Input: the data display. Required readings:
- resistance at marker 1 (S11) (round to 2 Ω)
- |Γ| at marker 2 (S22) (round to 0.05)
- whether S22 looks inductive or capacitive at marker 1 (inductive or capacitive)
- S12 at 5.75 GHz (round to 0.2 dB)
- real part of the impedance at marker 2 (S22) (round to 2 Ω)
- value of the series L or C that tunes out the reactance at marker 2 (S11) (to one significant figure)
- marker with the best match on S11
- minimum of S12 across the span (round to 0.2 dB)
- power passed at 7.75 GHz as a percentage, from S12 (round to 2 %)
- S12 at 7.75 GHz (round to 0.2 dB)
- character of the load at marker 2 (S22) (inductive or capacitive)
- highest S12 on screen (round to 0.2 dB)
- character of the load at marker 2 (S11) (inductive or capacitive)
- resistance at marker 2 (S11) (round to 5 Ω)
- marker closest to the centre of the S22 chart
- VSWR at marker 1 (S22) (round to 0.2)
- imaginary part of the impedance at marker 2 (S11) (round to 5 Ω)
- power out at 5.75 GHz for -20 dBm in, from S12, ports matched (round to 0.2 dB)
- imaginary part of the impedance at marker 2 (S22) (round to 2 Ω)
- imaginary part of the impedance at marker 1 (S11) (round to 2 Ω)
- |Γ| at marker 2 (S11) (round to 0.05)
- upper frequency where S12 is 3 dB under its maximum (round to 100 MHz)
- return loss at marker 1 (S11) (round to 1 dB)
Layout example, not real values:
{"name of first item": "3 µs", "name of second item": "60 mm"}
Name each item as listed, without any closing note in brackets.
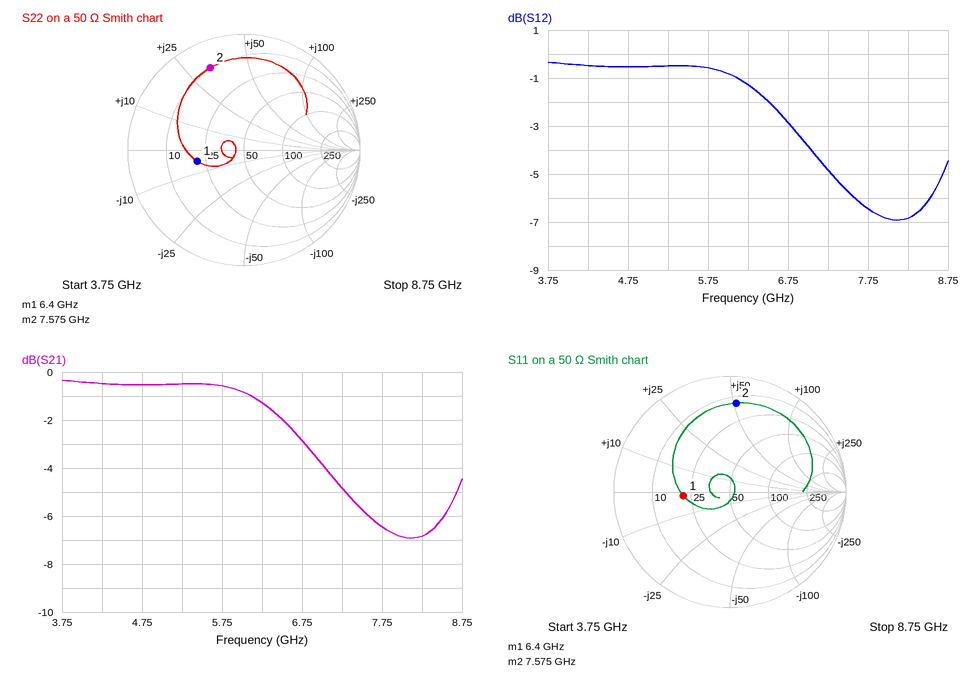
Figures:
{"resistance at marker 1 (S11)": "22 Ω", "|Γ| at marker 2 (S22)": "0.75", "whether S22 looks inductive or capacitive at marker 1": "capacitive", "S12 at 5.75 GHz": "-0.6 dB", "real part of the impedance at marker 2 (S22)": "10 Ω", "value of the series L or C that tunes out the reactance at marker 2 (S11)": "400 fF", "marker with the best match on S11": "marker 1", "minimum of S12 across the span": "-7.0 dB", "power passed at 7.75 GHz as a percentage, from S12": "22 %", "S12 at 7.75 GHz": "-6.4 dB", "character of the load at marker 2 (S22)": "inductive", "highest S12 on screen": "-0.4 dB", "character of the load at marker 2 (S11)": "inductive", "resistance at marker 2 (S11)": "15 Ω", "marker closest to the centre of the S22 chart": "marker 1", "VSWR at marker 1 (S22)": "2.4", "imaginary part of the impedance at marker 2 (S11)": "+50 Ω", "power out at 5.75 GHz for -20 dBm in, from S12, ports matched": "-20.6 dBm", "imaginary part of the impedance at marker 2 (S22)": "+32 Ω", "imaginary part of the impedance at marker 1 (S11)": "-2 Ω", "|Γ| at marker 2 (S11)": "0.75", "upper frequency where S12 is 3 dB under its maximum": "6.9 GHz", "return loss at marker 1 (S11)": "8 dB"}
